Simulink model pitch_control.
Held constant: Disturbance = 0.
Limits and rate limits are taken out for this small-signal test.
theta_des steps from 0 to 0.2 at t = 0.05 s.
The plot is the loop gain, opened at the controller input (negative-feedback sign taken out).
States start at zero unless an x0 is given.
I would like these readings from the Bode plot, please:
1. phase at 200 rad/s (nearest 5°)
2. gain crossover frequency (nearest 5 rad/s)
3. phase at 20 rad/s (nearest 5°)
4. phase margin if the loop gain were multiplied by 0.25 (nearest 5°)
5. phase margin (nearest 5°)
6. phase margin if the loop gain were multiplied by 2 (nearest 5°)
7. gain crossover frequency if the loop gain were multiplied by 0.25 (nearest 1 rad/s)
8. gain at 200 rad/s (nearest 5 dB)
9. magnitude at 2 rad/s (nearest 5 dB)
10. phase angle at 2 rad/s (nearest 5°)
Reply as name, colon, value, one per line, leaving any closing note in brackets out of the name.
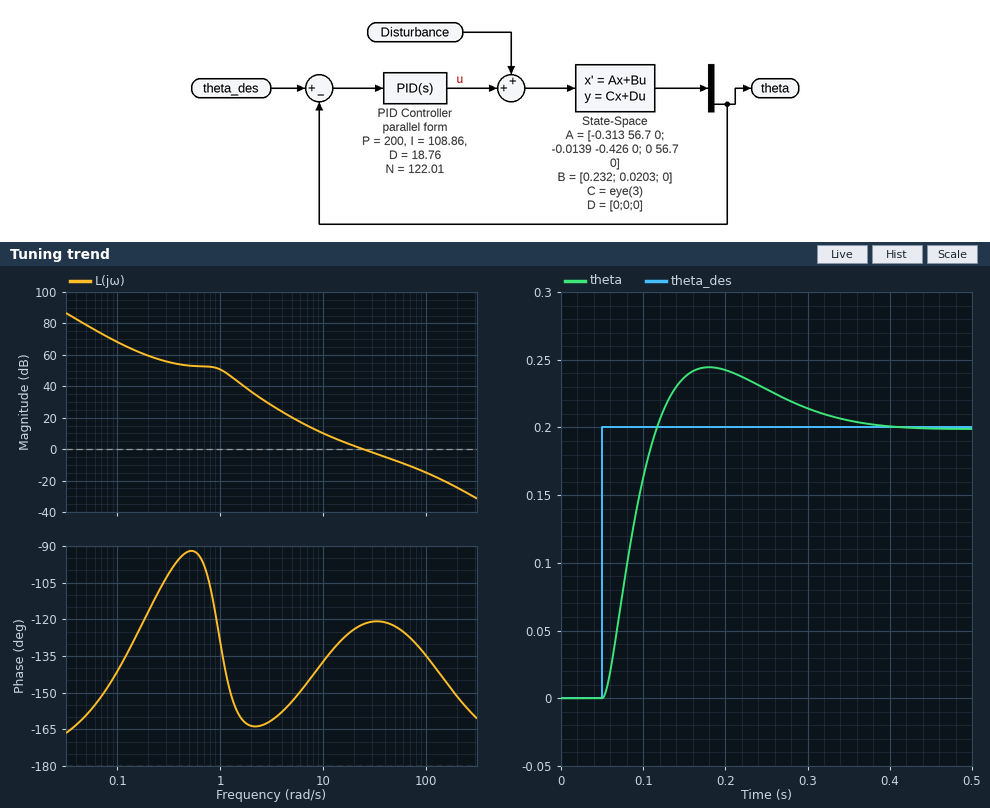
phase at 200 rad/s: -150°
gain crossover frequency: 25 rad/s
phase at 20 rad/s: -125°
phase margin if the loop gain were multiplied by 0.25: 40°
phase margin: 60°
phase margin if the loop gain were multiplied by 2: 60°
gain crossover frequency if the loop gain were multiplied by 0.25: 9 rad/s
gain at 200 rad/s: -25 dB
magnitude at 2 rad/s: 35 dB
phase angle at 2 rad/s: -165°
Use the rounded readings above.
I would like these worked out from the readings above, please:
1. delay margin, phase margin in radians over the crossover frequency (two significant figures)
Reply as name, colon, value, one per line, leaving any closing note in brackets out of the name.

delay margin, phase margin in radians over the crossover frequency: 0.042 s
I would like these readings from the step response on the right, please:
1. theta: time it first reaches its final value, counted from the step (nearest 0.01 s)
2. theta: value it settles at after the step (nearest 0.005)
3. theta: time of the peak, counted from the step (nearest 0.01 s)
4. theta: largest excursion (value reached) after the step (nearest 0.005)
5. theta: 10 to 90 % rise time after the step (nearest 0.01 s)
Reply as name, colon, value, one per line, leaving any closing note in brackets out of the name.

theta: time it first reaches its final value, counted from the step: 0.07 s
theta: value it settles at after the step: 0.200
theta: time of the peak, counted from the step: 0.13 s
theta: largest excursion (value reached) after the step: 0.245
theta: 10 to 90 % rise time after the step: 0.05 s
